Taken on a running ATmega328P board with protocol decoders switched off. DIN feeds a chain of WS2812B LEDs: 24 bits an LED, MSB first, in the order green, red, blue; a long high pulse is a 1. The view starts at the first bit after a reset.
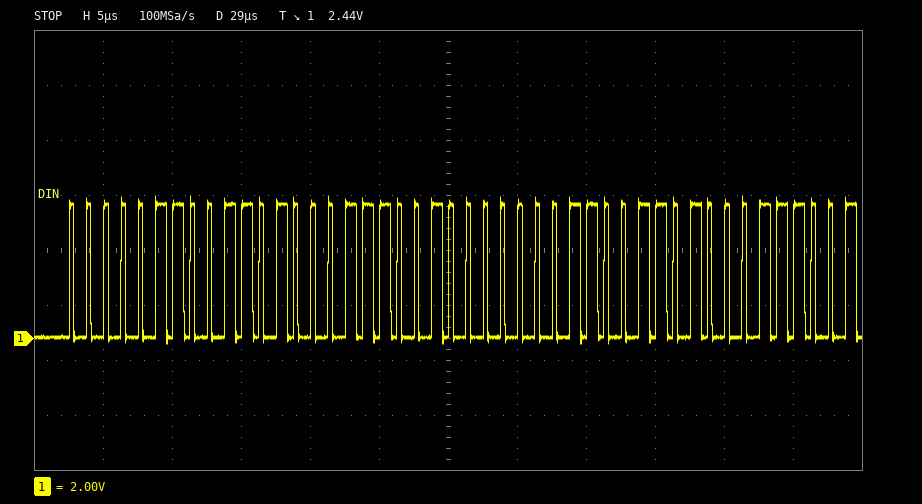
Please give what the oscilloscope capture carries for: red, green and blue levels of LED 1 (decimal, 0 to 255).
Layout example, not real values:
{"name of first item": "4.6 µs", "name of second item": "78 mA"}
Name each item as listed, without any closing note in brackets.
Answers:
{"red, green and blue levels of LED 1": "104, 6, 228"}
